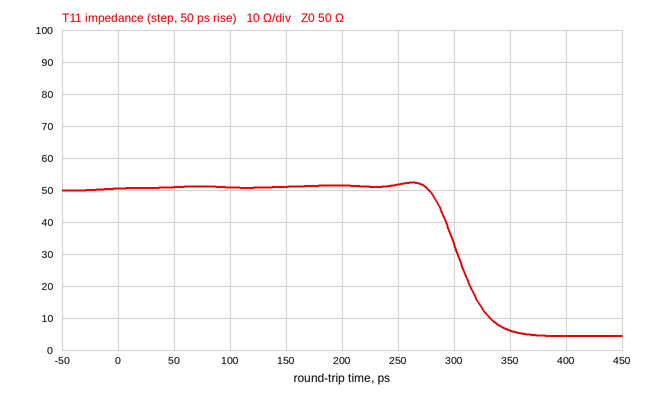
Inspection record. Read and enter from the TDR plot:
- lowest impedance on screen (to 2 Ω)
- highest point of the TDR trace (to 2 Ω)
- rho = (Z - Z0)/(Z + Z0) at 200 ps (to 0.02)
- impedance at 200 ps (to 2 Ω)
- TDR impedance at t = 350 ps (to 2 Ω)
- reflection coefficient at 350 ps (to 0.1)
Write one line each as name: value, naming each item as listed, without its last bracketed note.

lowest impedance on screen: 4 Ω
highest point of the TDR trace: 52 Ω
rho = (Z - Z0)/(Z + Z0) at 200 ps: +0.02
impedance at 200 ps: 52 Ω
TDR impedance at t = 350 ps: 6 Ω
reflection coefficient at 350 ps: -0.8
